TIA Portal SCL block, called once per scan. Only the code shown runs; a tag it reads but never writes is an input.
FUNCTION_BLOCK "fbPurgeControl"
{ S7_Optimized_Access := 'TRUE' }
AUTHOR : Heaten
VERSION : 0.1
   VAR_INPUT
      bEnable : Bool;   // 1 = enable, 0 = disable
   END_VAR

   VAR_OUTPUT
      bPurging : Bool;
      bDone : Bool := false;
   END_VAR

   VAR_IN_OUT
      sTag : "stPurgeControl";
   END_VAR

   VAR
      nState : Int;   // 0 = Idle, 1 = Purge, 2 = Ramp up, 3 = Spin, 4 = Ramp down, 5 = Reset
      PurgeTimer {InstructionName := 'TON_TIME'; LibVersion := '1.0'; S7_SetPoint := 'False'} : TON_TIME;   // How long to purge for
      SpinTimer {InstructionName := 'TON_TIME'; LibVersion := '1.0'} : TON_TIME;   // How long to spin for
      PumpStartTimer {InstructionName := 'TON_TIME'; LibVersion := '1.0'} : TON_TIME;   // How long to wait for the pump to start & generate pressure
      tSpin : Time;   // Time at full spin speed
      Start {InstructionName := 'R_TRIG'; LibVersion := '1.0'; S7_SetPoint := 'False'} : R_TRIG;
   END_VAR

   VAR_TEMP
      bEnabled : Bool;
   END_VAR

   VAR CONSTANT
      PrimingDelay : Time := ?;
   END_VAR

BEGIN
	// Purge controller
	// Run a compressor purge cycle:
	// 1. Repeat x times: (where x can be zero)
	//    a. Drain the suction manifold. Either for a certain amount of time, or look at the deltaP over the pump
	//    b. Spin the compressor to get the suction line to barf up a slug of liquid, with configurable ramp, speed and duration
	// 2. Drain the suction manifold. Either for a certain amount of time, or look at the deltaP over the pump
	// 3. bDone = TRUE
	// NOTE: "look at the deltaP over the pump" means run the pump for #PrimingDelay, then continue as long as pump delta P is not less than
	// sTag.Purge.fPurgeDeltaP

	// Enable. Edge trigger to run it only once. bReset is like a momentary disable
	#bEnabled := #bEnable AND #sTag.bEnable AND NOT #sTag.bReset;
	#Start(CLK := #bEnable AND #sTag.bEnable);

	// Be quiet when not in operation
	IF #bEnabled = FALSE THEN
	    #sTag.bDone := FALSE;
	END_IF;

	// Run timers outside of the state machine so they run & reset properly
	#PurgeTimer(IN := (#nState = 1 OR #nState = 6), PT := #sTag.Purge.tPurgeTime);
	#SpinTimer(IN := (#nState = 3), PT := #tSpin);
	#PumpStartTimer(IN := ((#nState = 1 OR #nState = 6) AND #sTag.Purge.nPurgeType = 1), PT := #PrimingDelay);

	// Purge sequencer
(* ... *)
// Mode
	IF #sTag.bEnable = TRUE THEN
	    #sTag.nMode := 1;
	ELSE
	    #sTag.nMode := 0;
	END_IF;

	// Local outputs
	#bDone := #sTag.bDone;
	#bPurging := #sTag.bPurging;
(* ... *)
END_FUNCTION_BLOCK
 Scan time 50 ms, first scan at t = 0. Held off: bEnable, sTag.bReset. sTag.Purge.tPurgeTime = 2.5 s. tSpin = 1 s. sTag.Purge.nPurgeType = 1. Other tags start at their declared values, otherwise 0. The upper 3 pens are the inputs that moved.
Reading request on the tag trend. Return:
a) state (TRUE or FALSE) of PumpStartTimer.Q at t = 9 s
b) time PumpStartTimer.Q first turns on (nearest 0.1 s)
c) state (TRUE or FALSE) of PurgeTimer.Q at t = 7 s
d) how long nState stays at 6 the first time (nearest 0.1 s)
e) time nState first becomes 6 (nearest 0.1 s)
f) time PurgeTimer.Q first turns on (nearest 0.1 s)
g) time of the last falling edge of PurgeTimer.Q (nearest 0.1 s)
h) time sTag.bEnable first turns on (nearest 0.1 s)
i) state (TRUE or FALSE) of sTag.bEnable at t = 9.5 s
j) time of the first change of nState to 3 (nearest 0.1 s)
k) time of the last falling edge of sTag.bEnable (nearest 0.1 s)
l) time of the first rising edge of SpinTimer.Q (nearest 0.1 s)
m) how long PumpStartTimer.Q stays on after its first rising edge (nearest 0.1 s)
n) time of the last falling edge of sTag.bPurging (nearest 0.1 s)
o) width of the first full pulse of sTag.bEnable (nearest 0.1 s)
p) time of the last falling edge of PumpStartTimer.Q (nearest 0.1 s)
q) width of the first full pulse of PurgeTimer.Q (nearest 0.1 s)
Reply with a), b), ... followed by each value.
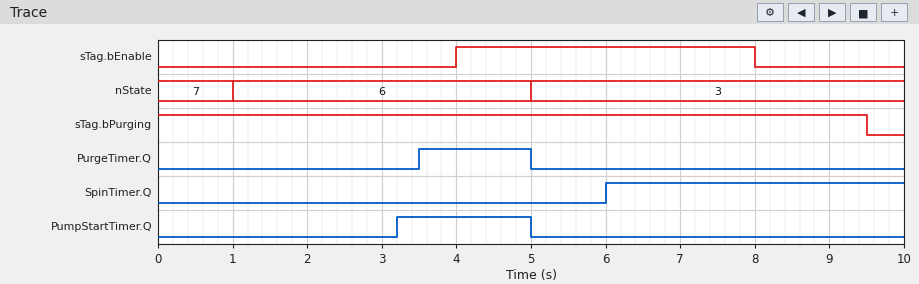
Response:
a) FALSE
b) 3.2 s
c) FALSE
d) 4.0 s
e) 1.0 s
f) 3.5 s
g) 5.0 s
h) 4.0 s
i) FALSE
j) 5.0 s
k) 8.0 s
l) 6.0 s
m) 1.8 s
n) 9.5 s
o) 4.0 s
p) 5.0 s
q) 1.5 s
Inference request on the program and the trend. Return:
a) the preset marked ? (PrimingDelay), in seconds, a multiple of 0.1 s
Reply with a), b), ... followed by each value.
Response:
a) 2.2 s
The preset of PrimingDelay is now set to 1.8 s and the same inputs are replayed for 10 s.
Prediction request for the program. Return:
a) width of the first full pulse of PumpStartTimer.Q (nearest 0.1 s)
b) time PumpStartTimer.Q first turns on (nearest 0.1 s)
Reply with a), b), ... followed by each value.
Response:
a) 2.2 s
b) 2.8 s
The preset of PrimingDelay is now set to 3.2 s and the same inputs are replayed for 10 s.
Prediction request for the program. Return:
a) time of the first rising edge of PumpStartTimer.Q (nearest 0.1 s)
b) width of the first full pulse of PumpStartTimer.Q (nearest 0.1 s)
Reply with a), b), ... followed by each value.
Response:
a) 4.2 s
b) 0.8 s
